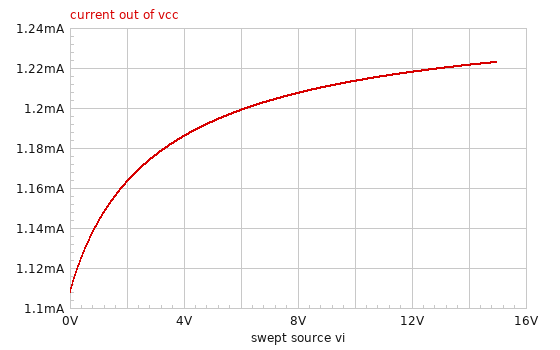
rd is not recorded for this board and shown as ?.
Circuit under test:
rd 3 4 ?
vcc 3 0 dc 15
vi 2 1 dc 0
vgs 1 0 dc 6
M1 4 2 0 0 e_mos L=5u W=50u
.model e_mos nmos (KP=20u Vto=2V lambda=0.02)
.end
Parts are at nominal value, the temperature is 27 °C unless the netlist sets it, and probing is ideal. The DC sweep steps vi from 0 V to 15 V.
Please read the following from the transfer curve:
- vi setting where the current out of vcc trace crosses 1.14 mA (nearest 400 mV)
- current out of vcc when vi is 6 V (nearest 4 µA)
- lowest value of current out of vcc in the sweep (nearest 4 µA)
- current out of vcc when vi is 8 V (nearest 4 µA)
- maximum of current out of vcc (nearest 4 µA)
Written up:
800 mV
1.200 mA
1.108 mA
1.208 mA
1.224 mA
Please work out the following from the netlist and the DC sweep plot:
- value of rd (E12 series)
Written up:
12 kΩ
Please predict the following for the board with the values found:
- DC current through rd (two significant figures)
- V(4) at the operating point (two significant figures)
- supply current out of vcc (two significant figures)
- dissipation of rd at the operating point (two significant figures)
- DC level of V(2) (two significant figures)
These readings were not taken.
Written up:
1.1 mA
1.7 V
1.1 mA
15 mW
6.0 V
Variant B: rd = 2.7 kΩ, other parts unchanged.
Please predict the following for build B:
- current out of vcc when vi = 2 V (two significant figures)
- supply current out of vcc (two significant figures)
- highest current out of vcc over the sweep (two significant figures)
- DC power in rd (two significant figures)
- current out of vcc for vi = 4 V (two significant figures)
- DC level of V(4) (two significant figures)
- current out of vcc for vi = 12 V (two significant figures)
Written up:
3.8 mA
1.9 mA
5.1 mA
9.9 mW
4.4 mA
9.8 V
5.0 mA
